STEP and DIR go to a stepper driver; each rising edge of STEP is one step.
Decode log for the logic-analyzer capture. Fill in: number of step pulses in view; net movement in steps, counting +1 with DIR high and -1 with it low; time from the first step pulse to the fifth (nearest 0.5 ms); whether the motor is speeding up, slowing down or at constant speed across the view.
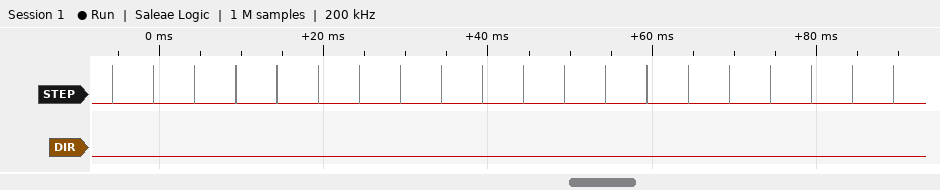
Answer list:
20
-20
20.0 ms
constant speed
